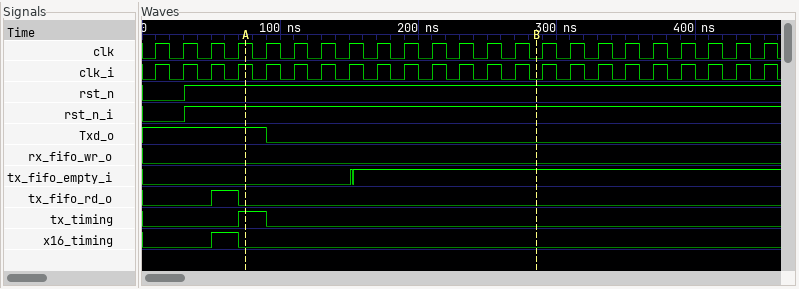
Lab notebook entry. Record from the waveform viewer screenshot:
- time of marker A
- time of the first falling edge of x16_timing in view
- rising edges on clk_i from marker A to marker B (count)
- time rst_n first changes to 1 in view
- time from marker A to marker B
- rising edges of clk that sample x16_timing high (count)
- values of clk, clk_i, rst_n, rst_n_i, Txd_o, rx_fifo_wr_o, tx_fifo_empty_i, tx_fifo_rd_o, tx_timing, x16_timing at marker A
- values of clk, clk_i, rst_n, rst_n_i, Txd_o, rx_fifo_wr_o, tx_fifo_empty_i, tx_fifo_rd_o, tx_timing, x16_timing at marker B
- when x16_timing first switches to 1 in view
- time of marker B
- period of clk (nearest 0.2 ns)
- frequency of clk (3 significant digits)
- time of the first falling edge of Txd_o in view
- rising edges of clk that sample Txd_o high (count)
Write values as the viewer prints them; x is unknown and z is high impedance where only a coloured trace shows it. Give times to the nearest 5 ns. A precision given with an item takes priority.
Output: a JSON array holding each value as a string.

["75 ns", "70 ns", "10", "30 ns", "210 ns", "1", "clk=1, clk_i=1, rst_n=1, rst_n_i=1, Txd_o=1, rx_fifo_wr_o=0, tx_fifo_empty_i=0, tx_fifo_rd_o=0, tx_timing=1, x16_timing=0", "clk=0, clk_i=0, rst_n=1, rst_n_i=1, Txd_o=0, rx_fifo_wr_o=0, tx_fifo_empty_i=1, tx_fifo_rd_o=0, tx_timing=0, x16_timing=0", "50 ns", "285 ns", "20 ns", "50.0 MHz", "90 ns", "5"]
